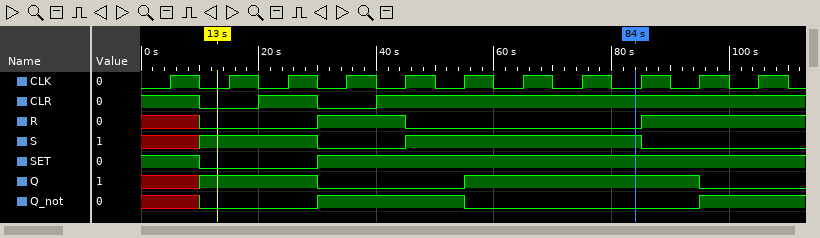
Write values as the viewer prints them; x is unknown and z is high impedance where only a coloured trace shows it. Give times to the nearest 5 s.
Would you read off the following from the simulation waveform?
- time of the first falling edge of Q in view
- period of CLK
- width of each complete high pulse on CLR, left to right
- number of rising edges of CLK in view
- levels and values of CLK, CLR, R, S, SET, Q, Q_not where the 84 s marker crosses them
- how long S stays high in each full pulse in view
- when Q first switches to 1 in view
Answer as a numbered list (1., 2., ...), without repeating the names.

1. 30 s
2. 10 s
3. 10 s
4. 11
5. CLK=0, CLR=1, R=0, S=1, SET=1, Q=1, Q_not=0
6. 40 s
7. 10 s
